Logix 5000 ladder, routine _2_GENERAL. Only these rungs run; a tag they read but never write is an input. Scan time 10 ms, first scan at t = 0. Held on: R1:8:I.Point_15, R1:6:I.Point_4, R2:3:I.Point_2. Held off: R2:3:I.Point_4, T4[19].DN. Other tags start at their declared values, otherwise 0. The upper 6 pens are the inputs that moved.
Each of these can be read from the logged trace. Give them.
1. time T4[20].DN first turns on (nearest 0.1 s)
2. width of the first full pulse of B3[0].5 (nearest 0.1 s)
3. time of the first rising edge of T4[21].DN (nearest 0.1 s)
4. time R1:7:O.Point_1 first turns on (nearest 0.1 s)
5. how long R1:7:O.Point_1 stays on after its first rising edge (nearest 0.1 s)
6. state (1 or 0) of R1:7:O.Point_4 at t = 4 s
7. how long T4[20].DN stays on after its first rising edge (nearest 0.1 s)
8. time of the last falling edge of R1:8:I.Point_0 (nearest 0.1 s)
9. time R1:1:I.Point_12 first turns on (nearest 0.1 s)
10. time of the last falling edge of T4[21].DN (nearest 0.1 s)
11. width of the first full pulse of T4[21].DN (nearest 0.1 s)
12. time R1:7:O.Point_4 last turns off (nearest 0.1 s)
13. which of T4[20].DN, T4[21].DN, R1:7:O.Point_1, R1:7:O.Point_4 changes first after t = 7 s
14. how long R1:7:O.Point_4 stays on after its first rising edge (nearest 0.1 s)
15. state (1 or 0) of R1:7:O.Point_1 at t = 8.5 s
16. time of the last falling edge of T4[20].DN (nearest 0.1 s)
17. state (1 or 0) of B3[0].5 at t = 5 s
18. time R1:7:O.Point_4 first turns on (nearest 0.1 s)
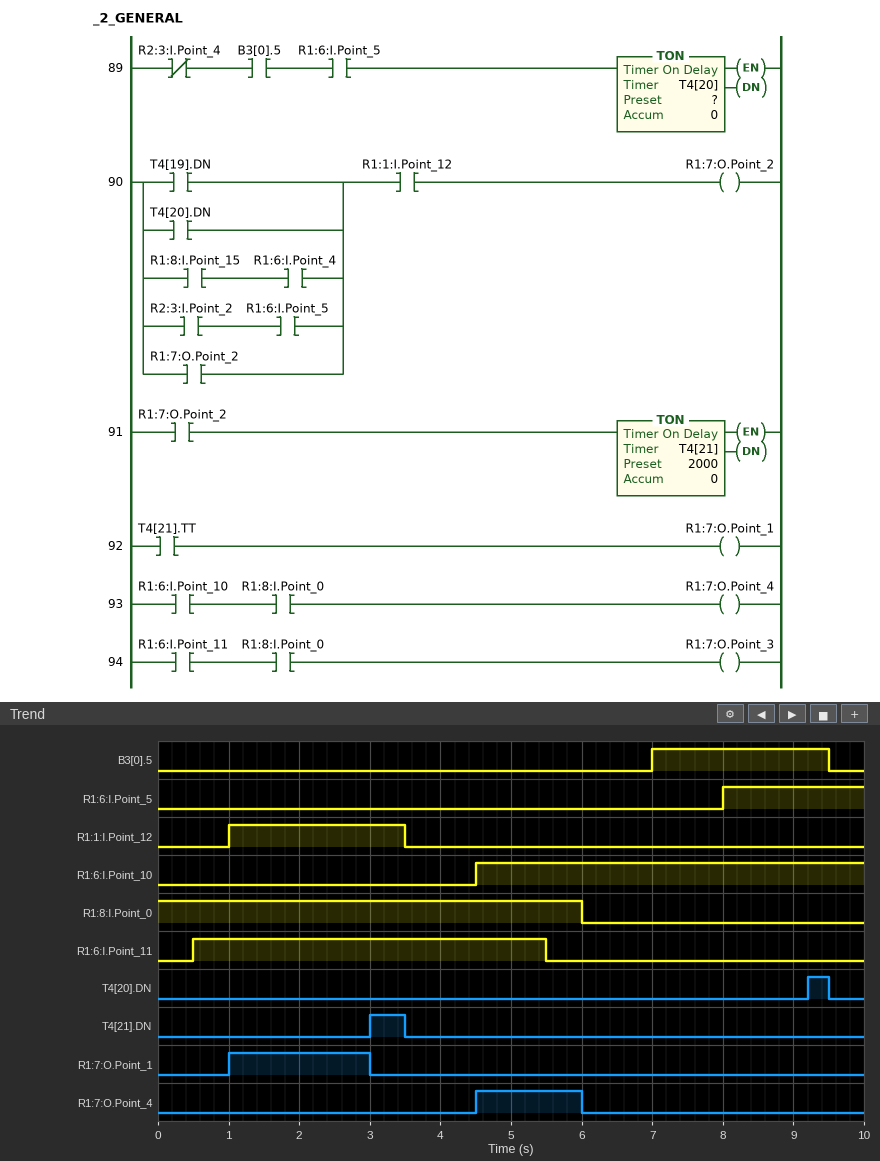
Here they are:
9.2 s
2.5 s
3.0 s
1.0 s
2.0 s
0
0.3 s
6.0 s
1.0 s
3.5 s
0.5 s
6.0 s
T4[20].DN
1.5 s
0
9.5 s
0
4.5 s
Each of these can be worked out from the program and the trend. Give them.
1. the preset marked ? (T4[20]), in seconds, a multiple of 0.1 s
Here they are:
1.2 s
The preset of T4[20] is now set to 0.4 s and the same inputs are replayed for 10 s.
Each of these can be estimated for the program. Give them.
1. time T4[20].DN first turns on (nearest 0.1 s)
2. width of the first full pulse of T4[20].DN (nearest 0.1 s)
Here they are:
8.4 s
1.1 s
